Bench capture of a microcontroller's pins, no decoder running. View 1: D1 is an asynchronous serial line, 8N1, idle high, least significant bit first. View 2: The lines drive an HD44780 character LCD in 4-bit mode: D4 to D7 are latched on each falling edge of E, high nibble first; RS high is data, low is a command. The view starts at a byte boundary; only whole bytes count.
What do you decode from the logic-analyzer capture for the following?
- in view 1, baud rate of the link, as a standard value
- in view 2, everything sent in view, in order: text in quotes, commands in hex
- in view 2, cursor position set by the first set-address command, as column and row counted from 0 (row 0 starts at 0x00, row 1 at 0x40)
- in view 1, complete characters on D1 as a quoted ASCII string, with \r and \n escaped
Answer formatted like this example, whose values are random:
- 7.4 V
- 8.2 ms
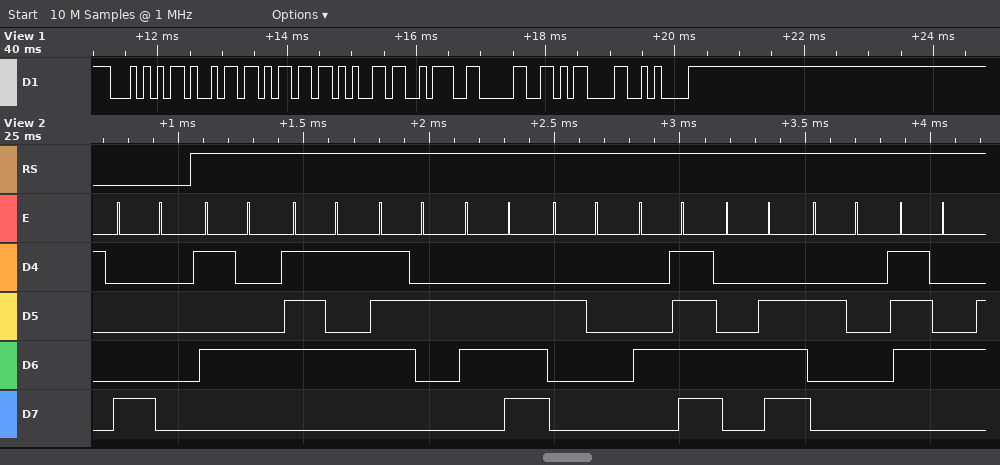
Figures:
- 9600 baud
- 0x80 "Turn ON t"
- column 0, row 0
- "Time:0\r\n"
